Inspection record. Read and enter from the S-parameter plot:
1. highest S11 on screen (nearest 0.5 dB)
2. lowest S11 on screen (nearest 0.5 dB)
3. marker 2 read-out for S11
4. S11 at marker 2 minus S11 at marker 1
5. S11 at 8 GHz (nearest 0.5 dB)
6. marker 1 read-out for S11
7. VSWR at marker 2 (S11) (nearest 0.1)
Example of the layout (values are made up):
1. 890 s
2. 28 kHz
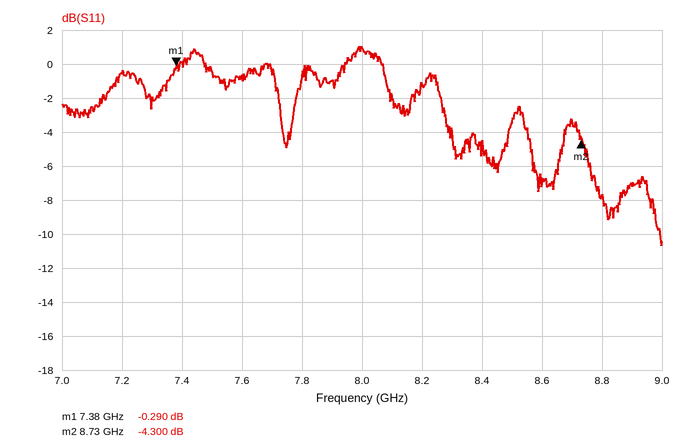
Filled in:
1. 1.0 dB
2. -10.5 dB
3. -4.300 dB
4. -4.010 dB
5. 1.0 dB
6. -0.290 dB
7. 4.1
